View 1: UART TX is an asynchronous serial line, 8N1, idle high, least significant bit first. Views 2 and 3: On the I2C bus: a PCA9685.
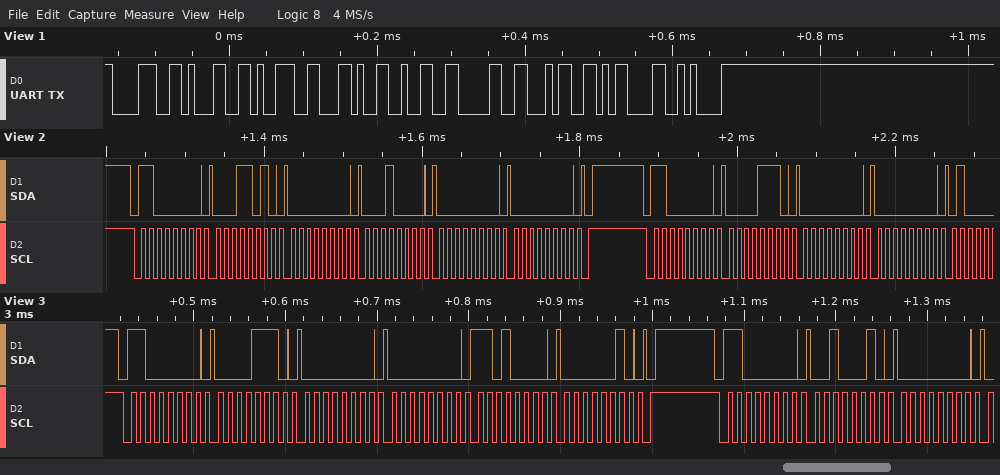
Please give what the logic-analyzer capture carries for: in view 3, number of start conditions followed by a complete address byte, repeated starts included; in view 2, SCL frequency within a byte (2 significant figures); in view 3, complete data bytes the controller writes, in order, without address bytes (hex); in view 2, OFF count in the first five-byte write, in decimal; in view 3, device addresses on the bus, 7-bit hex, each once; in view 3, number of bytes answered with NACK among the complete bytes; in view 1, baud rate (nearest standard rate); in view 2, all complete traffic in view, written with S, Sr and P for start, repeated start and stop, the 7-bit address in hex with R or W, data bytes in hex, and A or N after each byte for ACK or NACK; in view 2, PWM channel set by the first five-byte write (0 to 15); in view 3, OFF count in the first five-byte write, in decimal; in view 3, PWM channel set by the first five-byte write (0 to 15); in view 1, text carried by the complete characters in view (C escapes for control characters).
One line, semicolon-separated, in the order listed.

2; 100 kHz; 0E 00 00 D0 02 22 00; 0; 0x60; 0; 115200 baud; S 60W A 1A A 00 A 10 A 00 A 00 A P S 60W A 0E A 00 A 00 A; 5; 720; 2; "819,204\r\n"
